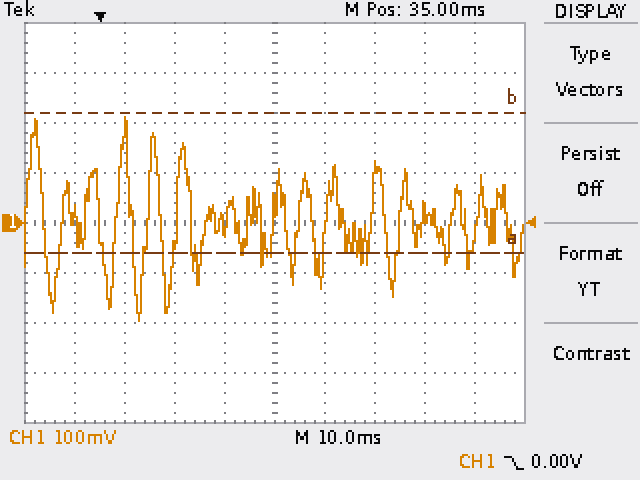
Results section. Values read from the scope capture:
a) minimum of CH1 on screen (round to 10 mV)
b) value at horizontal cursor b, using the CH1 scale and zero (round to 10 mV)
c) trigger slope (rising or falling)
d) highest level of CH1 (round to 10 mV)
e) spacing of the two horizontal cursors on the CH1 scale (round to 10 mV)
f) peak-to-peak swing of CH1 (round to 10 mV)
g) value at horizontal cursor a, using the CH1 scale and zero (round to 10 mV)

-200 mV
220 mV
falling
210 mV
280 mV
410 mV
-60 mV
